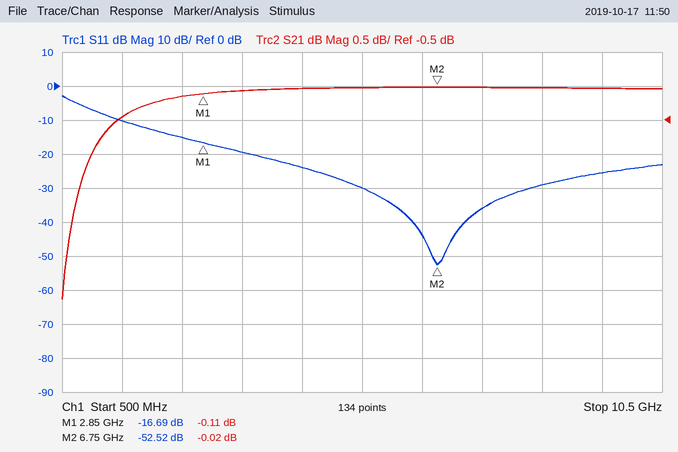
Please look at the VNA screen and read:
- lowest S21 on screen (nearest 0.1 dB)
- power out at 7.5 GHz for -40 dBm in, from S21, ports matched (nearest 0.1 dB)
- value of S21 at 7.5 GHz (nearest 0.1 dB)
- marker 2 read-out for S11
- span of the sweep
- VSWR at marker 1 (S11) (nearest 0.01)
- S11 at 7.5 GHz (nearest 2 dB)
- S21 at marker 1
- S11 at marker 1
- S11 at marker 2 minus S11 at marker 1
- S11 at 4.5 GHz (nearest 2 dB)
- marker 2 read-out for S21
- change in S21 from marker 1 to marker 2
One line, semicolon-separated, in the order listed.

-3.1 dB; -40.0 dBm; 0.0 dB; -52.52 dB; 10 GHz; 1.34; -36 dB; -0.11 dB; -16.69 dB; -35.83 dB; -24 dB; -0.02 dB; 0.09 dB
